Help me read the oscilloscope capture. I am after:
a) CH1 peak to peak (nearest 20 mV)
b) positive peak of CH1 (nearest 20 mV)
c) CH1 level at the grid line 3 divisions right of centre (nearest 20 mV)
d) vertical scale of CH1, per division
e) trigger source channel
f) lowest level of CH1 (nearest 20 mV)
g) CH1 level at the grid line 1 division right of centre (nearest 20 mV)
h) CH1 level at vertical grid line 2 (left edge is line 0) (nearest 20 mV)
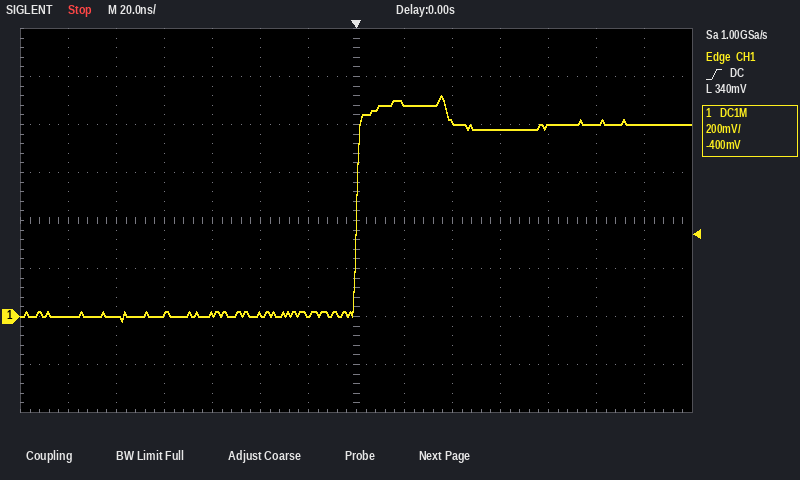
940 mV
920 mV
780 mV
200 mV
CH1
-20 mV
880 mV
0 mV
